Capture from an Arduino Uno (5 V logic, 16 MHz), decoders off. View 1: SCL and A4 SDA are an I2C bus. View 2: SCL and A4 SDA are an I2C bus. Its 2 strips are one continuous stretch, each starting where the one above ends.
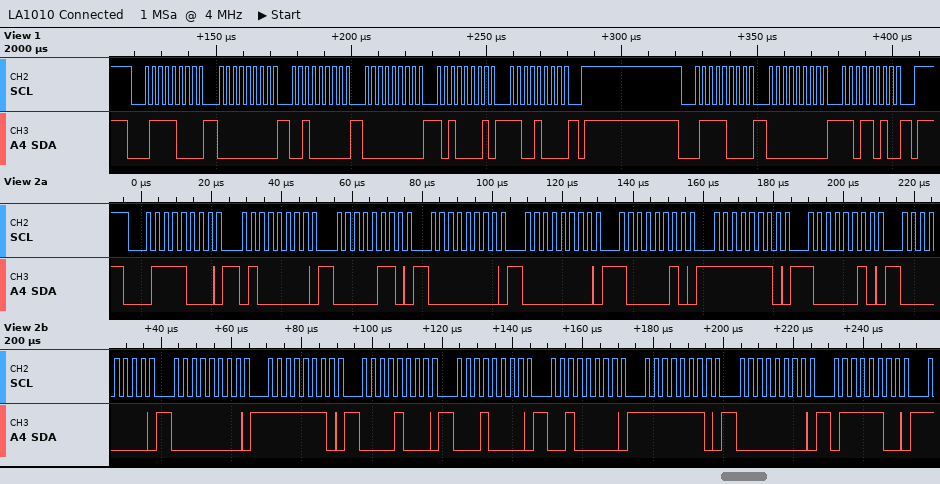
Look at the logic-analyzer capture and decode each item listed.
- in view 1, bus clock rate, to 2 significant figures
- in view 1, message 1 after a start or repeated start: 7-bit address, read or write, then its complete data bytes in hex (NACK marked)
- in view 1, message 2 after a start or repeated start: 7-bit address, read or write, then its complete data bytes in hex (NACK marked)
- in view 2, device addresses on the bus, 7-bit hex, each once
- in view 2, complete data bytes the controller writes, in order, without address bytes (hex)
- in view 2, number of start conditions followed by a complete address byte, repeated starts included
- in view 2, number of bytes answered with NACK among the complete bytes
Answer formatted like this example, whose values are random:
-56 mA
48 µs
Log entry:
400 kHz
0x3C write: 00 20 00 A1 C8
0x3C write: 00 DA
0x3C
40 06 00 00 82 FE 82 00 00 FE 08 10 20 FE 00 7C
1
0
